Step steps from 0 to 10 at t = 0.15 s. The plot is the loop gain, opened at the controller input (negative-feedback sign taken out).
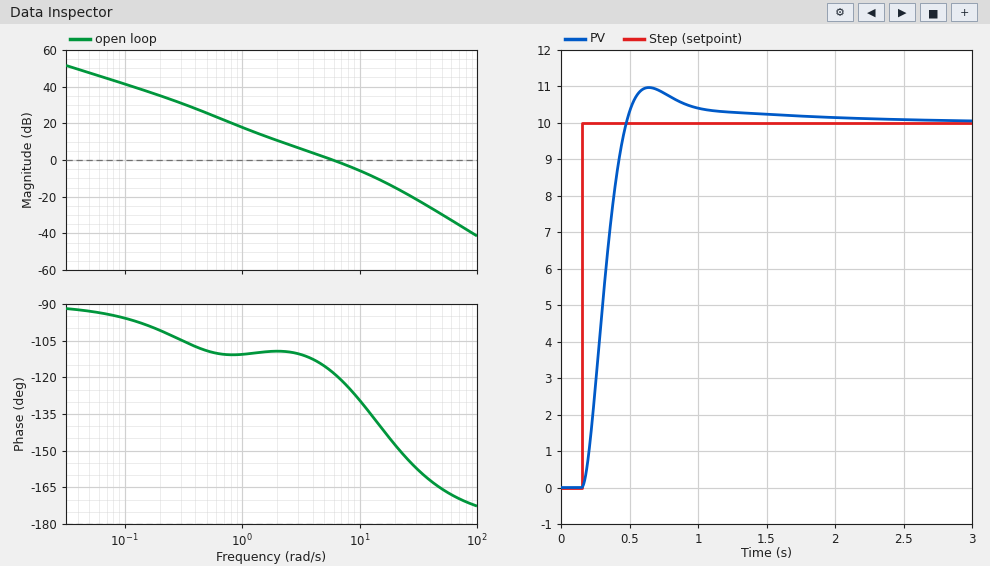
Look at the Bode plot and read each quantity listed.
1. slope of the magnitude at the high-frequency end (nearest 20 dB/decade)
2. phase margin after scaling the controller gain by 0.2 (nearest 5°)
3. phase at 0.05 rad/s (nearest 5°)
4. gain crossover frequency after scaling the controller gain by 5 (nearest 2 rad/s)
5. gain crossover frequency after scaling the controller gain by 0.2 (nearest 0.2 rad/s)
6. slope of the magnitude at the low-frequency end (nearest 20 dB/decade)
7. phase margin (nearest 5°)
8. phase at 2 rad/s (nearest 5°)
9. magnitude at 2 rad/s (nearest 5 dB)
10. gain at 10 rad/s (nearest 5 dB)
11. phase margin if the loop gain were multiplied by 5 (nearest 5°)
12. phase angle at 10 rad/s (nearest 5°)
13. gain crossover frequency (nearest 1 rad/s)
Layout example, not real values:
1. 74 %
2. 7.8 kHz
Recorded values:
1. -40 dB/decade
2. 70°
3. -95°
4. 18 rad/s
5. 1.4 rad/s
6. -20 dB/decade
7. 60°
8. -110°
9. 10 dB
10. -5 dB
11. 35°
12. -130°
13. 6 rad/s
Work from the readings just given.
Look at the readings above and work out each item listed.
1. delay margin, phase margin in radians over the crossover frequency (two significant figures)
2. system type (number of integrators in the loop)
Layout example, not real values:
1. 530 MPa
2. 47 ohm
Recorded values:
1. 0.17 s
2. 1
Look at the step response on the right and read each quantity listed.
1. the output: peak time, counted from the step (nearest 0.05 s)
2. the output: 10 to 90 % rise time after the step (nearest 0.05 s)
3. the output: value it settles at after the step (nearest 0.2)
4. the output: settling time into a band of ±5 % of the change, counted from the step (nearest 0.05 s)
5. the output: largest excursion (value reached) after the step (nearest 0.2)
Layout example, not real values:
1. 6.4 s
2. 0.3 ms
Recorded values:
1. 0.50 s
2. 0.20 s
3. 10.0
4. 0.75 s
5. 11.0
